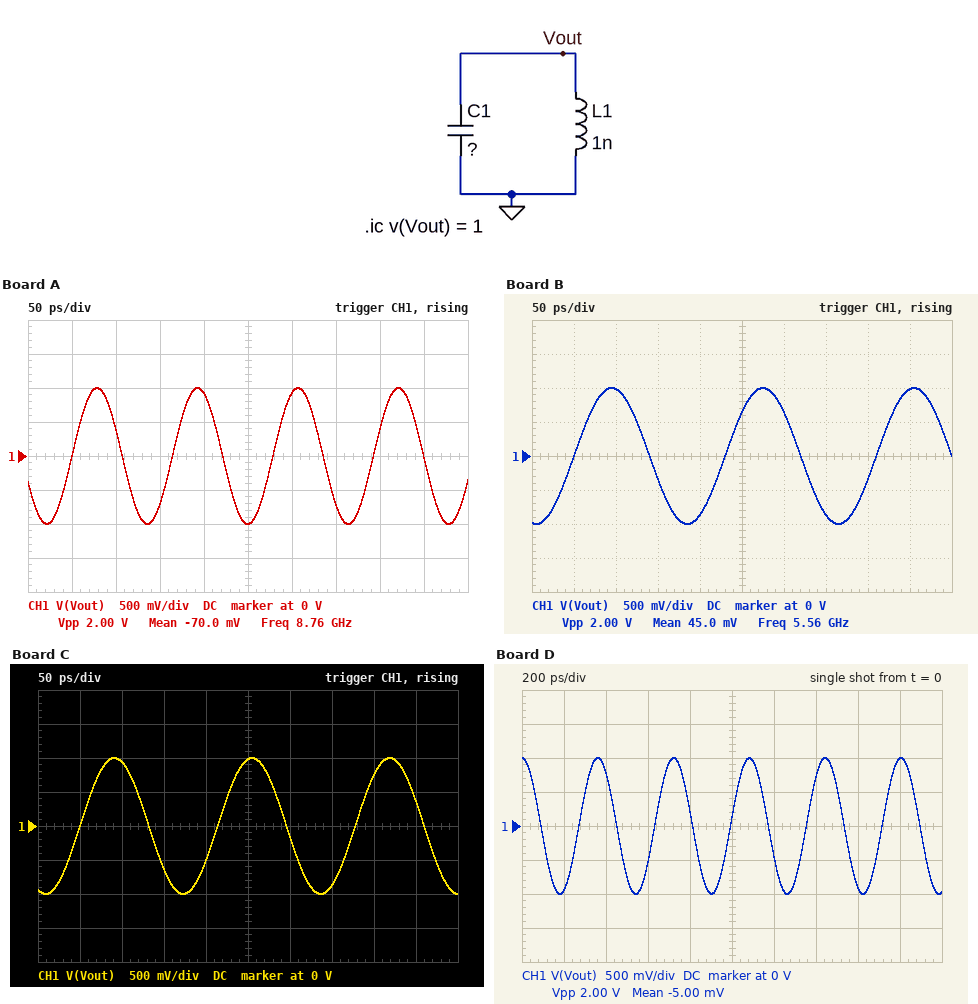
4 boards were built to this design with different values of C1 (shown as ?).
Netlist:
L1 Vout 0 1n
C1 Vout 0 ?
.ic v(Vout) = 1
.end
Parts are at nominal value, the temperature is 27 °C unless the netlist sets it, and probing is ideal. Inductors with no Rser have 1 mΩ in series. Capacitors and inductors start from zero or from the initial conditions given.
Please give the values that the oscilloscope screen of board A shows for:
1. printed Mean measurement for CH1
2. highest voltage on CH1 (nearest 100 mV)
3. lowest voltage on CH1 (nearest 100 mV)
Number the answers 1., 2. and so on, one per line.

1. -70.0 mV
2. 1.0 V
3. -1.0 V
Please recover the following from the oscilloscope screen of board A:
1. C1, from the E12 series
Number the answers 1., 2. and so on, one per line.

1. 330 fF
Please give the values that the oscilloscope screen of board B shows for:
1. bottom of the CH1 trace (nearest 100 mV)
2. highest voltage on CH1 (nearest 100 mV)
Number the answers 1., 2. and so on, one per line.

1. -1.0 V
2. 1.0 V
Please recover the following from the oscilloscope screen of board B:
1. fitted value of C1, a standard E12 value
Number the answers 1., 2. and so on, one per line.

1. 820 fF
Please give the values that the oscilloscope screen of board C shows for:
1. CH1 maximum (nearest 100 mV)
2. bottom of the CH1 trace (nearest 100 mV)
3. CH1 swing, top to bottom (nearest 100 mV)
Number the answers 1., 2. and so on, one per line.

1. 1.0 V
2. -1.0 V
3. 2.0 V
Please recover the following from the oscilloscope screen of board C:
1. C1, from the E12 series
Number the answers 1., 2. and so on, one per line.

1. 680 fF
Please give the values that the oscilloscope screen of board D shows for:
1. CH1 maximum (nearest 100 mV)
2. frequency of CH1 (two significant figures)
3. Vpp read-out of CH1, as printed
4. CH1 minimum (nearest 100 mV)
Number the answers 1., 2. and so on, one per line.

1. 1.0 V
2. 2.8 GHz
3. 2.00 V
4. -1.0 V
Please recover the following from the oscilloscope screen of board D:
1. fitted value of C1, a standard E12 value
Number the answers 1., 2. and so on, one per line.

1. 3.3 pF
